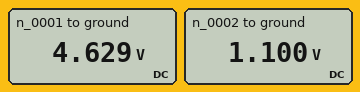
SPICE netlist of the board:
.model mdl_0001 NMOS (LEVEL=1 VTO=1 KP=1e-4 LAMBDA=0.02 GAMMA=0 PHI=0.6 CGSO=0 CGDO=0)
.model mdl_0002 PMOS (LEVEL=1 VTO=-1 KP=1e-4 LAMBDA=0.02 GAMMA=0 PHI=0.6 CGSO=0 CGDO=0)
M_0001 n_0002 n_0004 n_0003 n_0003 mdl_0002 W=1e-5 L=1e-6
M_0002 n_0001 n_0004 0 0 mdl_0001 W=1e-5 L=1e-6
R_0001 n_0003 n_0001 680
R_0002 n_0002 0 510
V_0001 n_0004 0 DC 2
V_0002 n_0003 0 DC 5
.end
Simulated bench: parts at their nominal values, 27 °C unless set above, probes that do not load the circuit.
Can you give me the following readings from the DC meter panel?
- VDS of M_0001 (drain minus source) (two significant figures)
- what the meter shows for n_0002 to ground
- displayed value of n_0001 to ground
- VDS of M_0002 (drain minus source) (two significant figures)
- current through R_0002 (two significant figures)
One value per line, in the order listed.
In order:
-3.9 V
1.100 V
4.629 V
4.6 V
2.2 mA
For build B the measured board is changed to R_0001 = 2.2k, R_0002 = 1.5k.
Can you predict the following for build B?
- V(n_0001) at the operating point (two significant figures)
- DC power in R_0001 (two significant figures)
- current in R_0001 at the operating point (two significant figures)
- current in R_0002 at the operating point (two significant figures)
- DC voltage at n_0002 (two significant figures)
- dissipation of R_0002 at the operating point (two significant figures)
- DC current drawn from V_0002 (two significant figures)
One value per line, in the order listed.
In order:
3.8 V
640 µW
540 µA
2.1 mA
3.1 V
6.4 mW
2.6 mA
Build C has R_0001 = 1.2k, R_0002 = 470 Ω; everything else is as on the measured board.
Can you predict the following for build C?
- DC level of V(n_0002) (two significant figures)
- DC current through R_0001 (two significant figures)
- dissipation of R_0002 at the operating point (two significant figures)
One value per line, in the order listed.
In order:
1.0 V
540 µA
2.2 mW
